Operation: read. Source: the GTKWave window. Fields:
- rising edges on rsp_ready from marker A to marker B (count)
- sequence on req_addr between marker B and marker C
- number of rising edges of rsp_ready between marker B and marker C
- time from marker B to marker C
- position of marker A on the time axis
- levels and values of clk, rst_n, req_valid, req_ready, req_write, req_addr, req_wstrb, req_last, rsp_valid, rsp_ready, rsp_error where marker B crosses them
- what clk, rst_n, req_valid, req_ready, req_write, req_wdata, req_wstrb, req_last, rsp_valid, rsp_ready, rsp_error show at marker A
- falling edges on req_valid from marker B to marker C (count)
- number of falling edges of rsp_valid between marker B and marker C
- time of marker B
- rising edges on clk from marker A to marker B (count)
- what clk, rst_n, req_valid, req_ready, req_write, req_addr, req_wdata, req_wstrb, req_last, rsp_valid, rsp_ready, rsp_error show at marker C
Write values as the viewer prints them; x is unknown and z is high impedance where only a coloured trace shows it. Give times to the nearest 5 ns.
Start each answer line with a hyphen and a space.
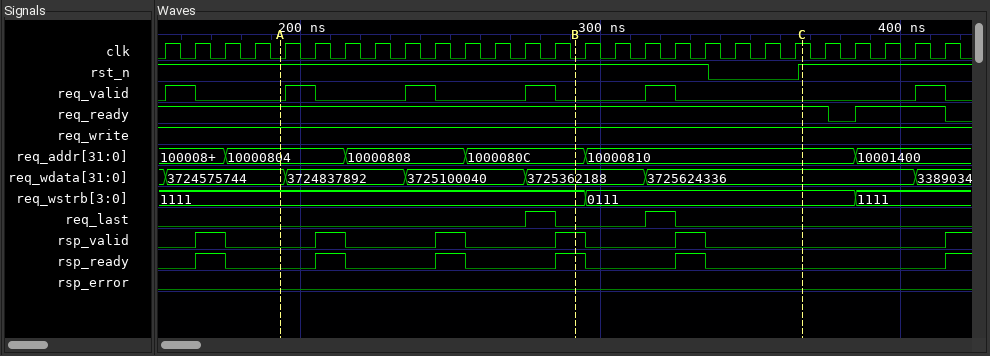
- 3
- 1000080C, 10000810
- 1
- 75 ns
- 195 ns
- clk=0, rst_n=1, req_valid=0, req_ready=1, req_write=1, req_addr=1000080C, req_wstrb=1111, req_last=0, rsp_valid=1, rsp_ready=1, rsp_error=0
- clk=0, rst_n=1, req_valid=0, req_ready=1, req_write=1, req_wdata=3724575744, req_wstrb=1111, req_last=0, rsp_valid=0, rsp_ready=0, rsp_error=0
- 1
- 2
- 290 ns
- 10
- clk=1, rst_n=1, req_valid=0, req_ready=1, req_write=1, req_addr=10000810, req_wdata=3725624336, req_wstrb=0111, req_last=0, rsp_valid=0, rsp_ready=0, rsp_error=0
